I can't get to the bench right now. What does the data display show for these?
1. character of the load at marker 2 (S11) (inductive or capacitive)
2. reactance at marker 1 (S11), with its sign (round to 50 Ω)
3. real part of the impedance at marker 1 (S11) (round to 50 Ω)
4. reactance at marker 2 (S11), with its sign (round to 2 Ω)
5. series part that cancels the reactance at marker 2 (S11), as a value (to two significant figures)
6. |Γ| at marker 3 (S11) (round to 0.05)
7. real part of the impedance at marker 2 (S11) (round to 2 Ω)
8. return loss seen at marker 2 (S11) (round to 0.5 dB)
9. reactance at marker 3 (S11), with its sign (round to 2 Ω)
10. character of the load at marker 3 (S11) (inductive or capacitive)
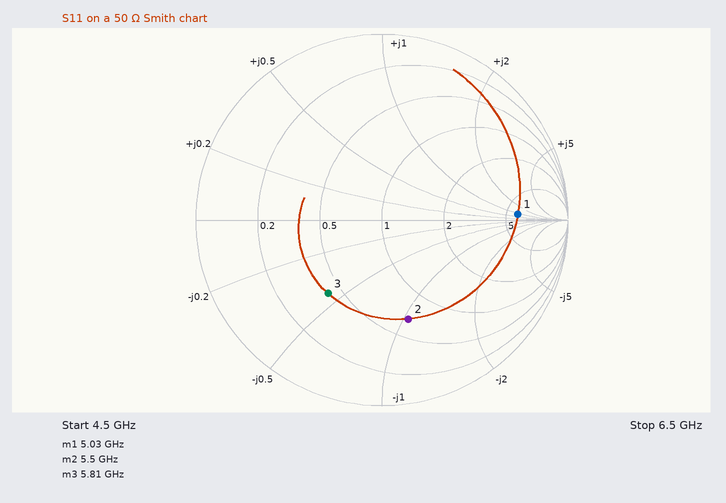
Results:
capacitive
+50 Ω
300 Ω
-52 Ω
1.5 nH
0.50
34 Ω
5.0 dB
-22 Ω
capacitive
